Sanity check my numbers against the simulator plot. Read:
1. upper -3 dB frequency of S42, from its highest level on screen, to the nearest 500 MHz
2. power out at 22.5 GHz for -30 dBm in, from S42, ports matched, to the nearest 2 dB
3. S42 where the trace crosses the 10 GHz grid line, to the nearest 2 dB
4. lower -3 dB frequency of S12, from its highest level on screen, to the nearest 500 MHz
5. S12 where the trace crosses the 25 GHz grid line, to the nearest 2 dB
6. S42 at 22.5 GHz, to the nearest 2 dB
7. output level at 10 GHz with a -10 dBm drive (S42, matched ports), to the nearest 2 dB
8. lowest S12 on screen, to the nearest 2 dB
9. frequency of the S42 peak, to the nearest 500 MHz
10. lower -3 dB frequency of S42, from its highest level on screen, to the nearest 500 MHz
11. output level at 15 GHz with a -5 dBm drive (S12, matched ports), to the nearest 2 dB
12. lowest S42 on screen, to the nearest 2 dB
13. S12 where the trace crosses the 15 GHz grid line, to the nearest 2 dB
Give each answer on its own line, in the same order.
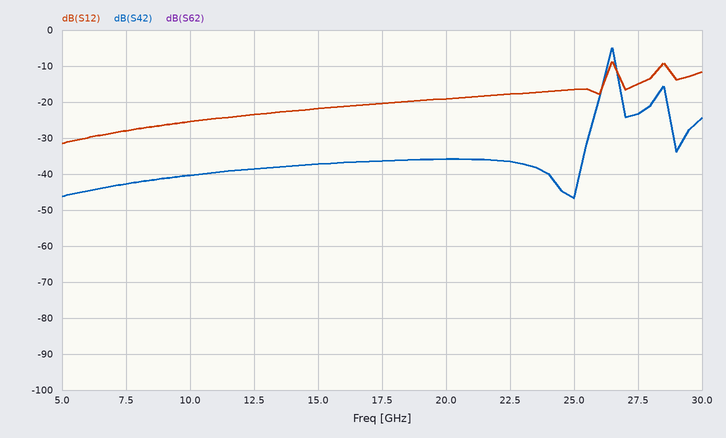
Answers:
26.5 GHz
-66 dBm
-40 dB
26.5 GHz
-16 dB
-36 dB
-50 dBm
-32 dB
26.5 GHz
26.5 GHz
-26 dBm
-46 dB
-22 dB
